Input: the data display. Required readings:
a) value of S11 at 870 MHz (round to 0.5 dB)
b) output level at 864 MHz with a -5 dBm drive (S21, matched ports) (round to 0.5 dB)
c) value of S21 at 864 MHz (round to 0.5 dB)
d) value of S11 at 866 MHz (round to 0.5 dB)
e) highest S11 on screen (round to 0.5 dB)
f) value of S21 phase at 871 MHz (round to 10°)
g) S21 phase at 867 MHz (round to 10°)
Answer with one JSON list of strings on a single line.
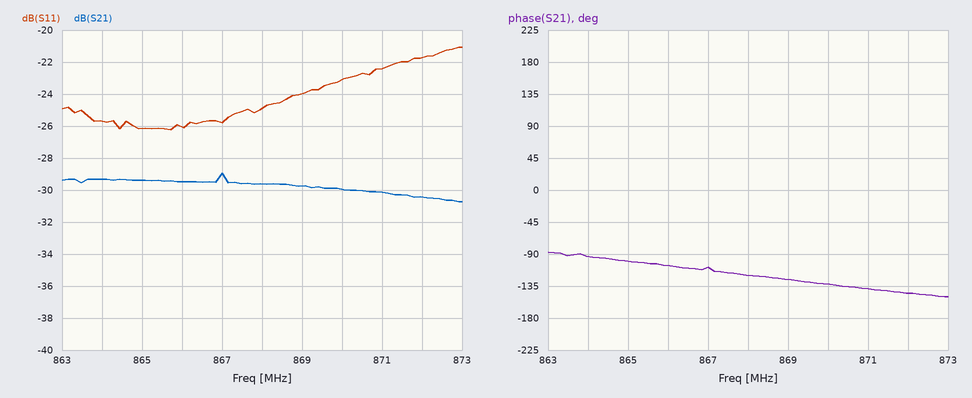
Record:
["-23.0 dB", "-34.5 dBm", "-29.5 dB", "-26.0 dB", "-21.0 dB", "-140°", "-110°"]
